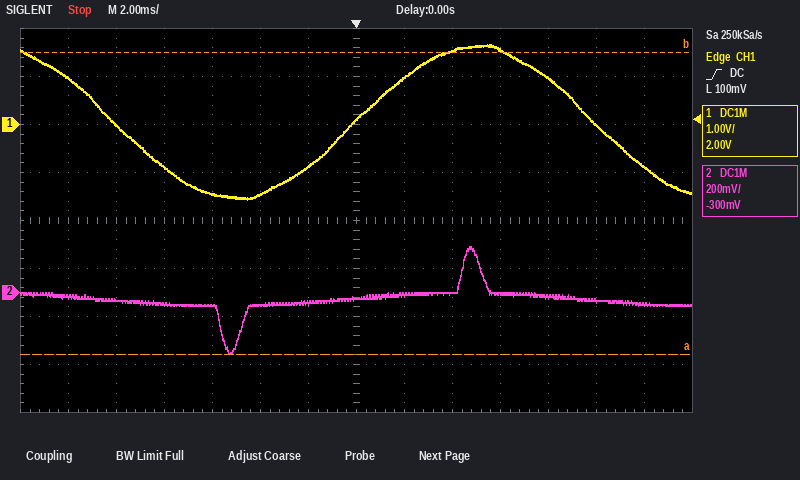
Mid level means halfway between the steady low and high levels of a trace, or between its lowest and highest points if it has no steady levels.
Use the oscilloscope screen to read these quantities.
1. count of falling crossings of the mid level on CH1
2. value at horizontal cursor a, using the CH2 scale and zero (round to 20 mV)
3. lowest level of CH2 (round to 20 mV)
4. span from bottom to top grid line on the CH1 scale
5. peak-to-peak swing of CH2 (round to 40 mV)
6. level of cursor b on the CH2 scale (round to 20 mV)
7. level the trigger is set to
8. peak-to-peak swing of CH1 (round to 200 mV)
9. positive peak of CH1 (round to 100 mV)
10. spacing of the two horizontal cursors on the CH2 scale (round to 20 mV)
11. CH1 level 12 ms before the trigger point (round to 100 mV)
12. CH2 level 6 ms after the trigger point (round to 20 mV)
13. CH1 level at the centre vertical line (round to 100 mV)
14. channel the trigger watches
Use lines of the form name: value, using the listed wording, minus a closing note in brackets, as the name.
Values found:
count of falling crossings of the mid level on CH1: 2
value at horizontal cursor a, using the CH2 scale and zero: -260 mV
lowest level of CH2: -260 mV
span from bottom to top grid line on the CH1 scale: 8 V
peak-to-peak swing of CH2: 440 mV
level of cursor b on the CH2 scale: 1.00 V
level the trigger is set to: 100 mV
peak-to-peak swing of CH1: 3.2 V
positive peak of CH1: 1.7 V
spacing of the two horizontal cursors on the CH2 scale: 1.26 V
CH1 level 12 ms before the trigger point: 1.0 V
CH2 level 6 ms after the trigger point: 0 mV
CH1 level at the centre vertical line: 100 mV
channel the trigger watches: CH1
